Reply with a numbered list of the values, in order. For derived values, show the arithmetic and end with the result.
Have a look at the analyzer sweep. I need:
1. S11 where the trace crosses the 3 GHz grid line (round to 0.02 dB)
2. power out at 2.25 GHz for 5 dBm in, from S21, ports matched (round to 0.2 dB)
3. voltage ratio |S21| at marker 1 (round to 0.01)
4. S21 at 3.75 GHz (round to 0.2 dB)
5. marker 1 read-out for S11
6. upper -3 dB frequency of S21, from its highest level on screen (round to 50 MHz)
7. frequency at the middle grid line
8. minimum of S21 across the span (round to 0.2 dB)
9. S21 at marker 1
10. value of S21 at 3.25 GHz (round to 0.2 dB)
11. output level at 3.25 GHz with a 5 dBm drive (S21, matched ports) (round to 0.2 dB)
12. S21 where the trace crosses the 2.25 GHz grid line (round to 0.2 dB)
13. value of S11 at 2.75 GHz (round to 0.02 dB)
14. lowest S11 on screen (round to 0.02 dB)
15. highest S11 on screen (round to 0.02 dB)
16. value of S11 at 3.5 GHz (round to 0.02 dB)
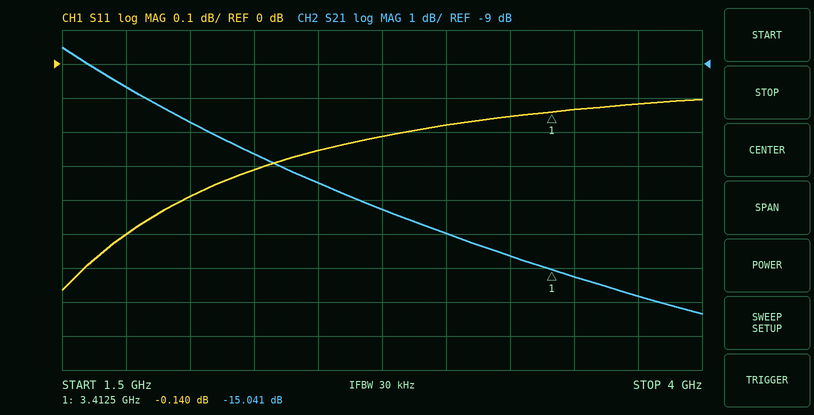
1. -0.18 dB
2. 5 dBm + (-11.6 dB) = -6.6 dBm
3. 10^(-15.041/20) ≈ 0.18
4. -15.8 dB
5. -0.140 dB
6. 2.20 GHz
7. 2.75 GHz
8. -16.4 dB
9. -15.041 dB
10. -14.6 dB
11. 5 dBm + (-14.6 dB) = -9.6 dBm
12. -11.6 dB
13. -0.22 dB
14. -0.66 dB
15. -0.10 dB
16. -0.14 dB
